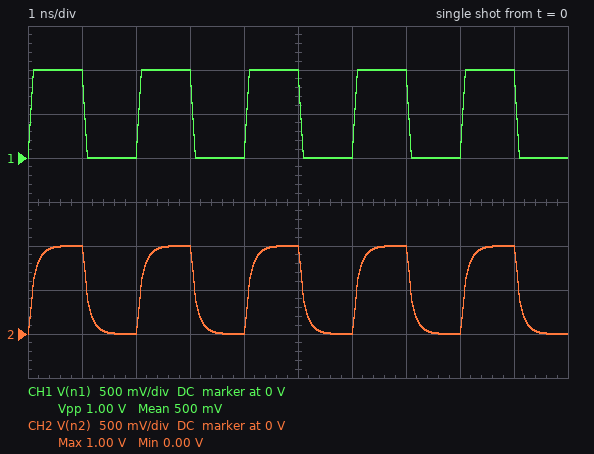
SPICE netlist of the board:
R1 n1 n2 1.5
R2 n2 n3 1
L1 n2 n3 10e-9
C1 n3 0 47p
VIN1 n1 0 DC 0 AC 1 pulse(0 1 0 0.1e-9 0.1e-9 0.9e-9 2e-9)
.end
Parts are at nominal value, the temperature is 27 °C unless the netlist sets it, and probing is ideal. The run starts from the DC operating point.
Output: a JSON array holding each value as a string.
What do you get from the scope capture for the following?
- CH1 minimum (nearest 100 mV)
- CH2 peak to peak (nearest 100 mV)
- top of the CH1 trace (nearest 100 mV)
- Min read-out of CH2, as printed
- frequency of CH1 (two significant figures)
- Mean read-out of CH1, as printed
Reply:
["0 V", "1.0 V", "1.0 V", "0.00 V", "500 MHz", "500 mV"]
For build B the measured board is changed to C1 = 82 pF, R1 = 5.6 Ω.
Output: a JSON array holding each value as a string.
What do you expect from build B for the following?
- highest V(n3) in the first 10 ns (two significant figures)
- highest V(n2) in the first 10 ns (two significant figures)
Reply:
["860 mV", "870 mV"]
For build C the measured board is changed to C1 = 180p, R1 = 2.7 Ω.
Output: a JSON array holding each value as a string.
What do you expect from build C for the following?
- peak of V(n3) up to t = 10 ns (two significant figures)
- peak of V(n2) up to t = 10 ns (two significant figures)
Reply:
["810 mV", "850 mV"]
